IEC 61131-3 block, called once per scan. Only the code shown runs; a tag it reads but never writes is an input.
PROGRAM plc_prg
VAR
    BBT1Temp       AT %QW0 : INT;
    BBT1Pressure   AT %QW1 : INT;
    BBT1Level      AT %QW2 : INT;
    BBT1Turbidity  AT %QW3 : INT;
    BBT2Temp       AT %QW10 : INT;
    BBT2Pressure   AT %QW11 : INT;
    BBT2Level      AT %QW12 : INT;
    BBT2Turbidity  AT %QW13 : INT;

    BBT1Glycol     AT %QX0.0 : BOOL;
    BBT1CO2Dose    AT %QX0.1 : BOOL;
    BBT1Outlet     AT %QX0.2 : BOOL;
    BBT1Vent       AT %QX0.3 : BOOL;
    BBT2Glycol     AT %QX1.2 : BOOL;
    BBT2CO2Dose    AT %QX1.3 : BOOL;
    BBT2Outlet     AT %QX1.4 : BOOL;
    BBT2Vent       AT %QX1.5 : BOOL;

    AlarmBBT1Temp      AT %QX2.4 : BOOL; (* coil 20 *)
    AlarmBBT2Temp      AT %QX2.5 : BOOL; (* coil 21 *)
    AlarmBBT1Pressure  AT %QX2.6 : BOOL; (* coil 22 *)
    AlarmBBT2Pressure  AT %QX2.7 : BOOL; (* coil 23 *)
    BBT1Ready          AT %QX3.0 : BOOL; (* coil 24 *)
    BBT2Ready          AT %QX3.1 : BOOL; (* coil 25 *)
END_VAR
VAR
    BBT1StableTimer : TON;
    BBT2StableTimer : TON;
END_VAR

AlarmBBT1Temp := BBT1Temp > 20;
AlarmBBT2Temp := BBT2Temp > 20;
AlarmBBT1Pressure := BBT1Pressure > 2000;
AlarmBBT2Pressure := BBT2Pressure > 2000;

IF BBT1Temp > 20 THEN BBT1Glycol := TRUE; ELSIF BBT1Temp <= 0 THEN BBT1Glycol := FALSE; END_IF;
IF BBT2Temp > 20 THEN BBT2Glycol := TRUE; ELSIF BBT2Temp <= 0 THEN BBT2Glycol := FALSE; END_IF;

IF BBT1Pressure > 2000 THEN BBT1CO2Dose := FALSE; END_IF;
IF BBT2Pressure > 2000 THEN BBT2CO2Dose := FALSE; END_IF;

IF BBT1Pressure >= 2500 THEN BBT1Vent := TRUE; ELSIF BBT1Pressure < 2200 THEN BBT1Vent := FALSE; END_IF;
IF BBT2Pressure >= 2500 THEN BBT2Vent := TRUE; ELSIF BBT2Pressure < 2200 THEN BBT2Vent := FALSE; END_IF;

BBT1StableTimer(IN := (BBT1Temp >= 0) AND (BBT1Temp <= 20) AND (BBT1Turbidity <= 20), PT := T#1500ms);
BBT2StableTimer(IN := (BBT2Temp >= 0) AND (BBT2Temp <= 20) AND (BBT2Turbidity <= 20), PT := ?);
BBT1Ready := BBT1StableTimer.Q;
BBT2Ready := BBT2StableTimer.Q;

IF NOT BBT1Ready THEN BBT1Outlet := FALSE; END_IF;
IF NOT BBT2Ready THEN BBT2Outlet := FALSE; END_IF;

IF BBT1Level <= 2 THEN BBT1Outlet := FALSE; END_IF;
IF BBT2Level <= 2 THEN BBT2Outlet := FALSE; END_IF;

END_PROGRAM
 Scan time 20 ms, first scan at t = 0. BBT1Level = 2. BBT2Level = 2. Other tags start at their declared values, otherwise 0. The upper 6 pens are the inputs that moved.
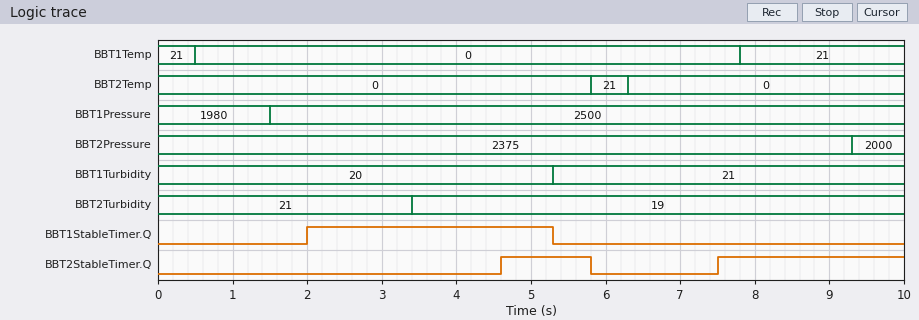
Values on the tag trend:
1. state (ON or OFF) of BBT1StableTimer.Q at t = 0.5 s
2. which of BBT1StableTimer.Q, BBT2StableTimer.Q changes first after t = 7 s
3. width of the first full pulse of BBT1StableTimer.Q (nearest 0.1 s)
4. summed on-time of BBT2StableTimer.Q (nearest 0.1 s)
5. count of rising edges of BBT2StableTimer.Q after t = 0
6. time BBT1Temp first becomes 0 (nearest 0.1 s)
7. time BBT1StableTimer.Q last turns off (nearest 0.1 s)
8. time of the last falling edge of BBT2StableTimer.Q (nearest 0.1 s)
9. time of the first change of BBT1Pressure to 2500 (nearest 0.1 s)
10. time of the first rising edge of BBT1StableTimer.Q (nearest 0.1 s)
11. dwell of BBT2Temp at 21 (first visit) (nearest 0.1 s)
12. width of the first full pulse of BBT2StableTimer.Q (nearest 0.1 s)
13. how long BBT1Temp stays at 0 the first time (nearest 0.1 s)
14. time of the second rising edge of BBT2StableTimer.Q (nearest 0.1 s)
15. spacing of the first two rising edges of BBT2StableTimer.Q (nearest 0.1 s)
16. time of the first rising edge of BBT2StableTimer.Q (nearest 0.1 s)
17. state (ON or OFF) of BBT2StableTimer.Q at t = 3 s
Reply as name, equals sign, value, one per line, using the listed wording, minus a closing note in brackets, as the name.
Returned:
state (ON or OFF) of BBT1StableTimer.Q at t = 0.5 s = OFF
which of BBT1StableTimer.Q, BBT2StableTimer.Q changes first after t = 7 s = BBT2StableTimer.Q
width of the first full pulse of BBT1StableTimer.Q = 3.3 s
summed on-time of BBT2StableTimer.Q = 3.7 s
count of rising edges of BBT2StableTimer.Q after t = 0 = 2
time BBT1Temp first becomes 0 = 0.5 s
time BBT1StableTimer.Q last turns off = 5.3 s
time of the last falling edge of BBT2StableTimer.Q = 5.8 s
time of the first change of BBT1Pressure to 2500 = 1.5 s
time of the first rising edge of BBT1StableTimer.Q = 2.0 s
dwell of BBT2Temp at 21 (first visit) = 0.5 s
width of the first full pulse of BBT2StableTimer.Q = 1.2 s
how long BBT1Temp stays at 0 the first time = 7.3 s
time of the second rising edge of BBT2StableTimer.Q = 7.5 s
spacing of the first two rising edges of BBT2StableTimer.Q = 2.9 s
time of the first rising edge of BBT2StableTimer.Q = 4.6 s
state (ON or OFF) of BBT2StableTimer.Q at t = 3 s = OFF
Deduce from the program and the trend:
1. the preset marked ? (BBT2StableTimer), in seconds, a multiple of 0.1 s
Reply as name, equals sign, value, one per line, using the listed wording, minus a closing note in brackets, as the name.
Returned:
the preset marked ? (BBT2StableTimer), in seconds, a multiple of 0.1 s = 1.2 s
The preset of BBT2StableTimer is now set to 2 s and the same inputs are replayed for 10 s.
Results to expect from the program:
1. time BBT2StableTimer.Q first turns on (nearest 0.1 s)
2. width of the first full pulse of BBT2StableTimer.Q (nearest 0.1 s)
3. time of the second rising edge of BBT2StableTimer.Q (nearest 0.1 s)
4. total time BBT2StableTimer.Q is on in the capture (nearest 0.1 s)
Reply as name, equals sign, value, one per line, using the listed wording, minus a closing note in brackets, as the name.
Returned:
time BBT2StableTimer.Q first turns on = 5.4 s
width of the first full pulse of BBT2StableTimer.Q = 0.4 s
time of the second rising edge of BBT2StableTimer.Q = 8.3 s
total time BBT2StableTimer.Q is on in the capture = 2.1 s
